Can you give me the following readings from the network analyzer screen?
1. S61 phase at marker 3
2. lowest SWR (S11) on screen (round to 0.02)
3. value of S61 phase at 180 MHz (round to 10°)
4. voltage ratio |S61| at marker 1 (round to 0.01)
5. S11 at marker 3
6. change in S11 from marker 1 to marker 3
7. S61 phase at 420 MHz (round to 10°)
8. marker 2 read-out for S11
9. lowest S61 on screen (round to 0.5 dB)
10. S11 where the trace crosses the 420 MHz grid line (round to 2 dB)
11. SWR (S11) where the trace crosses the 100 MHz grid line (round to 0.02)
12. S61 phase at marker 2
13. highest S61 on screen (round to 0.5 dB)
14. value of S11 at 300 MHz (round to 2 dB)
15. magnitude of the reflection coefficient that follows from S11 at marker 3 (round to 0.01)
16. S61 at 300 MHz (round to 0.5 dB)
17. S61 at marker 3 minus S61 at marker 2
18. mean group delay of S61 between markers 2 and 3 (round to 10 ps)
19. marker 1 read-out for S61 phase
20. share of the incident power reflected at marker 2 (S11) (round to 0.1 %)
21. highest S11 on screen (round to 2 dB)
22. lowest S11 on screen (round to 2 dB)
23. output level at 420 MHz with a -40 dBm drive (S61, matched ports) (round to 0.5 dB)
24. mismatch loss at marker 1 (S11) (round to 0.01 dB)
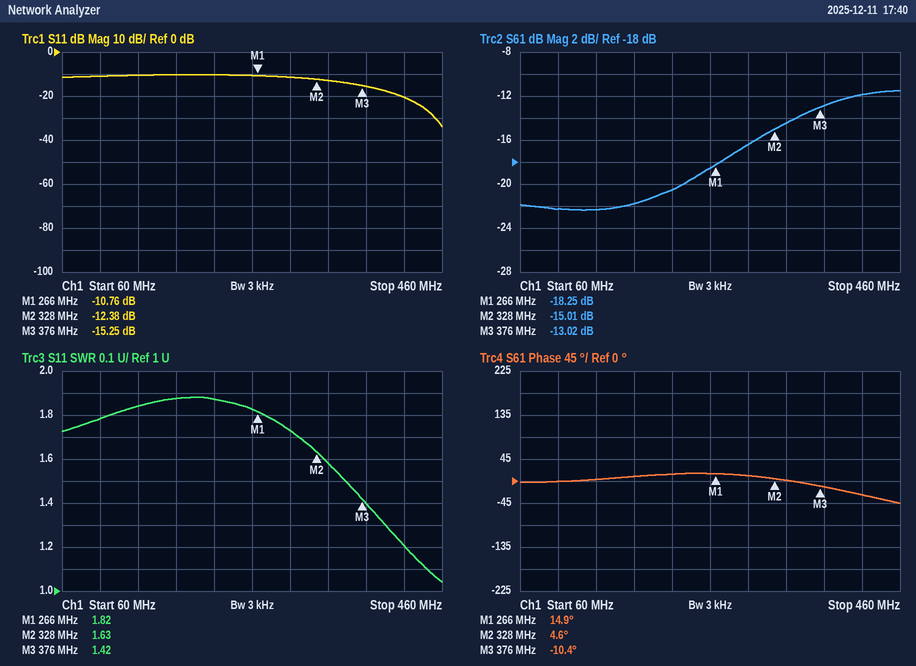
-10.4°
1.04
10°
0.12
-15.25 dB
-4.49 dB
-30°
-12.38 dB
-22.5 dB
-20 dB
1.78
4.6°
-11.5 dB
-12 dB
0.17
-16.5 dB
1.99 dB
870 ps
14.9°
5.8 %
-10 dB
-34 dB
-52.0 dBm
0.38 dB
